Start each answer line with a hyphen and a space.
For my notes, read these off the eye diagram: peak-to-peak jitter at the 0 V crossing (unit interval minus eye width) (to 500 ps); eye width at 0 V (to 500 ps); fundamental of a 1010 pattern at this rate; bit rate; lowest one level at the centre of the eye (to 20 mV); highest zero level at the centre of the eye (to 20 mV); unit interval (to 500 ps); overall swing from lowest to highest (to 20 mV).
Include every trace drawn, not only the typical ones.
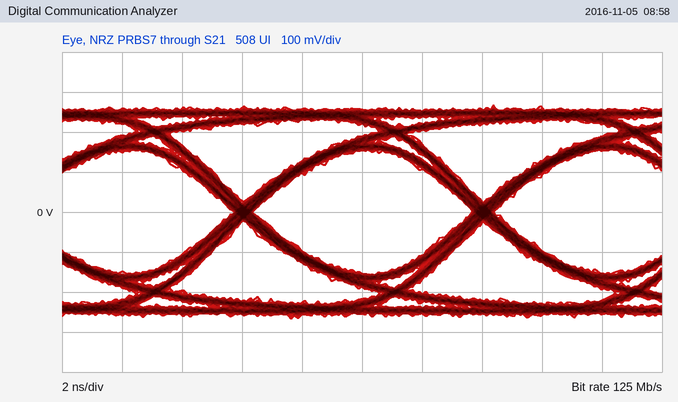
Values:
- 500 ps
- 7.5 ns
- 62.5 MHz
- 125 Mb/s
- 160 mV
- -160 mV
- 8.0 ns
- 540 mV
